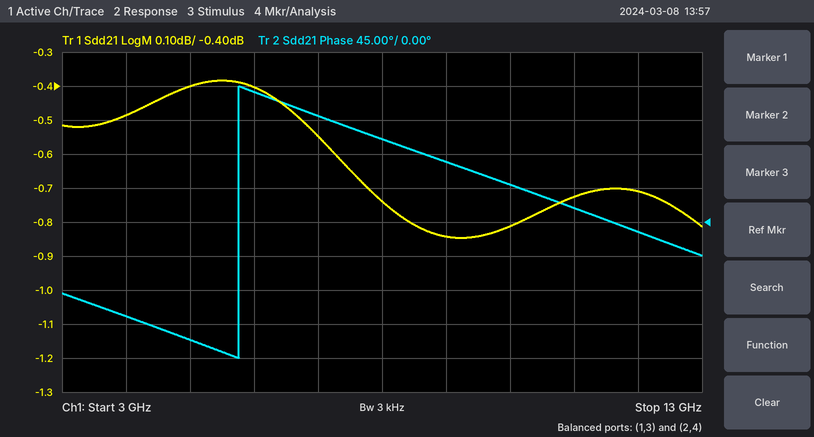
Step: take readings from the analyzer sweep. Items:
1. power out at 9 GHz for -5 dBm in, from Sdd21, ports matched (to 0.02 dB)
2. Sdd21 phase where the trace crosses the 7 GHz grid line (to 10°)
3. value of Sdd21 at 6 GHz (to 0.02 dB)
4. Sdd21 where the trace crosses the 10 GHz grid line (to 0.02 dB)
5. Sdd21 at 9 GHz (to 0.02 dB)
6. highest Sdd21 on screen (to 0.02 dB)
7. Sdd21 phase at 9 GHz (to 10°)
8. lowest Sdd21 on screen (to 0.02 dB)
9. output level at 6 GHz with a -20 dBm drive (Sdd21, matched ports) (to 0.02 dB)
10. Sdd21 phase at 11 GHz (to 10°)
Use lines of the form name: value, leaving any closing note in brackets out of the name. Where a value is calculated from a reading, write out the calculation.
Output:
power out at 9 GHz for -5 dBm in, from Sdd21, ports matched: -5 dBm + (-0.84 dB) = -5.84 dBm
Sdd21 phase where the trace crosses the 7 GHz grid line: 140°
value of Sdd21 at 6 GHz: -0.40 dB
Sdd21 where the trace crosses the 10 GHz grid line: -0.82 dB
Sdd21 at 9 GHz: -0.84 dB
highest Sdd21 on screen: -0.38 dB
Sdd21 phase at 9 GHz: 80°
lowest Sdd21 on screen: -0.84 dB
output level at 6 GHz with a -20 dBm drive (Sdd21, matched ports): -20 dBm + (-0.40 dB) = -20.40 dBm
Sdd21 phase at 11 GHz: 20°
